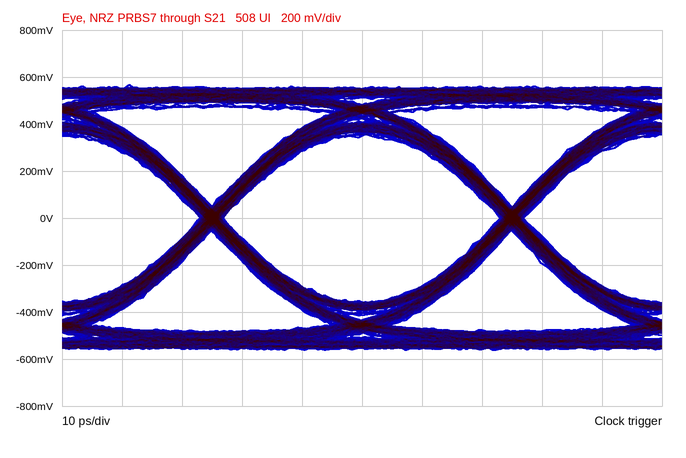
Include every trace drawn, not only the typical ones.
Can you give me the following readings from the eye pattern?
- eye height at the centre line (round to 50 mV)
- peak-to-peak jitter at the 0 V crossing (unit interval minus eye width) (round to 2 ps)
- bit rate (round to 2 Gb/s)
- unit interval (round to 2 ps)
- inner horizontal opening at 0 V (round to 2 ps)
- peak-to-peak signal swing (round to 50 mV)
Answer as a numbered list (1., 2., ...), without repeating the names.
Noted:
1. 700 mV
2. 4 ps
3. 20 Gb/s
4. 50 ps
5. 46 ps
6. 1.15 V
